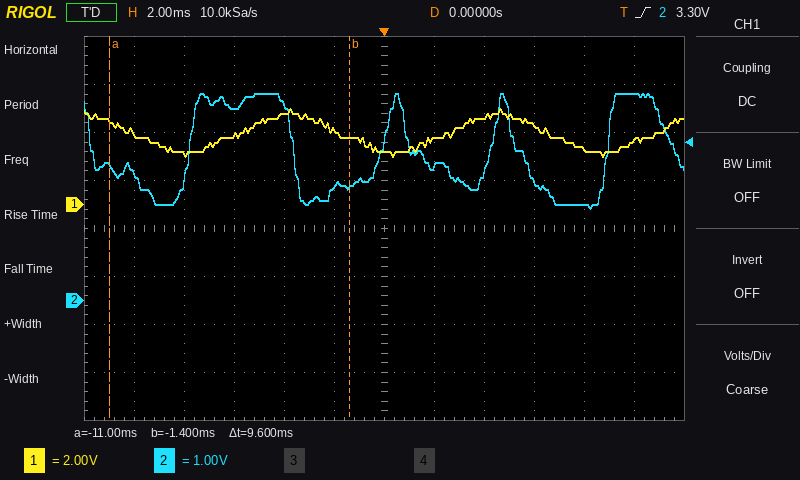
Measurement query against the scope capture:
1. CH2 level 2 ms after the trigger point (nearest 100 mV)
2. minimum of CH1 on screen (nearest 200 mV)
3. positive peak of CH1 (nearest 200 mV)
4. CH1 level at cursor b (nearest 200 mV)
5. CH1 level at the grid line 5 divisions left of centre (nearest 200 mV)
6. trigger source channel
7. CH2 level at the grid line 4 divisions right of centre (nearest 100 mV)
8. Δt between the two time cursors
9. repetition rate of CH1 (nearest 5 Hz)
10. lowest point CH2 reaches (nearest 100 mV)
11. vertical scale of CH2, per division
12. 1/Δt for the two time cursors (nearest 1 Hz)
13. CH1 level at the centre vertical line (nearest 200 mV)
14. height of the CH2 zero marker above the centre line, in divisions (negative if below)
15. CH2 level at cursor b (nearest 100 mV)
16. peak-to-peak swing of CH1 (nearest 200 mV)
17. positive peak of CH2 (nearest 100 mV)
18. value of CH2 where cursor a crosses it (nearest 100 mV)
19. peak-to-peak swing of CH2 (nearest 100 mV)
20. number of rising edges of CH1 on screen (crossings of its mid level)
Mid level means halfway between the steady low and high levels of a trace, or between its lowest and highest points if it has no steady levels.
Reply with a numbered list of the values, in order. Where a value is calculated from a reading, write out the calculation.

1. 2.8 V
2. 2.0 V
3. 4.0 V
4. 2.8 V
5. 3.0 V
6. CH2
7. 2.0 V
8. 9.6 ms
9. 120 Hz
10. 1.9 V
11. 1 V
12. 1 / 9.6 ms ≈ 104 Hz
13. 2.2 V
14. -1.5 div
15. 2.4 V
16. 4.0 V − (2.0 V) = 2.0 V
17. 4.3 V
18. 2.8 V
19. 4.3 V − (1.9 V) = 2.4 V
20. 3
